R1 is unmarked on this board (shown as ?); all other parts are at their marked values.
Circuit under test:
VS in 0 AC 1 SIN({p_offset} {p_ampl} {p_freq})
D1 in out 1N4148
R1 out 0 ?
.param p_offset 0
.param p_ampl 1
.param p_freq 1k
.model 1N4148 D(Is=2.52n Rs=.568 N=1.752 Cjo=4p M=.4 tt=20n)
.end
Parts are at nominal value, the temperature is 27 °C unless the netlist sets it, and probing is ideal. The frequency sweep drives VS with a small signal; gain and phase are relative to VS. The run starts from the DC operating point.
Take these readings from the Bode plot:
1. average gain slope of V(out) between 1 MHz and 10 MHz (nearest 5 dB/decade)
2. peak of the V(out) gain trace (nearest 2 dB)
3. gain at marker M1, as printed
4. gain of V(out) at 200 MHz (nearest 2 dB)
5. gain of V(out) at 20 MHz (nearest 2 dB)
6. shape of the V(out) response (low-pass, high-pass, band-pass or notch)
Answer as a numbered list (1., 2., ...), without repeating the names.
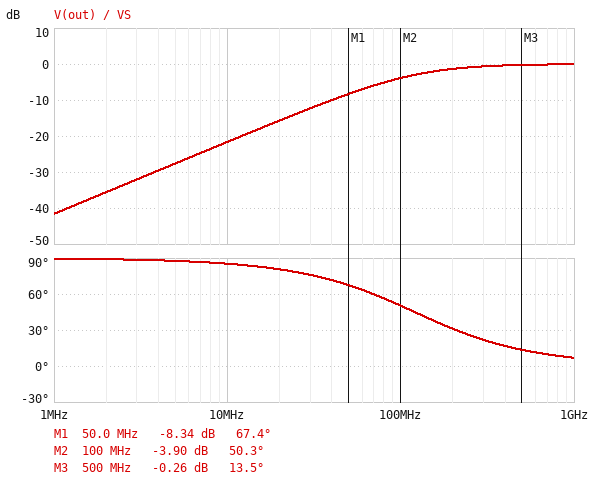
1. 20 dB/decade
2. 0 dB
3. -8.34 dB
4. -2 dB
5. -16 dB
6. high-pass
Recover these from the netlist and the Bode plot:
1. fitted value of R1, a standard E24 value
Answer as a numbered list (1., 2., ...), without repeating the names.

1. 330 Ω
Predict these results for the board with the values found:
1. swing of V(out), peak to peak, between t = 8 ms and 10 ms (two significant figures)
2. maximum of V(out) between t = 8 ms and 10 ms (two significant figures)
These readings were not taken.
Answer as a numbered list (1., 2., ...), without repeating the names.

1. 410 mV
2. 410 mV
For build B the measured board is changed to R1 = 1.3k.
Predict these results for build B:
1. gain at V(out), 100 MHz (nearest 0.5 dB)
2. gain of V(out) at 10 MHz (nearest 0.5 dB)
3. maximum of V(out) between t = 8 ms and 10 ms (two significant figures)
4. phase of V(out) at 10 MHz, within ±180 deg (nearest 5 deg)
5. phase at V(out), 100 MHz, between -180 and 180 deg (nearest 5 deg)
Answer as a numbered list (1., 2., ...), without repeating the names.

1. -0.5 dB
2. -10.0 dB
3. 460 mV
4. 70 deg
5. 15 deg
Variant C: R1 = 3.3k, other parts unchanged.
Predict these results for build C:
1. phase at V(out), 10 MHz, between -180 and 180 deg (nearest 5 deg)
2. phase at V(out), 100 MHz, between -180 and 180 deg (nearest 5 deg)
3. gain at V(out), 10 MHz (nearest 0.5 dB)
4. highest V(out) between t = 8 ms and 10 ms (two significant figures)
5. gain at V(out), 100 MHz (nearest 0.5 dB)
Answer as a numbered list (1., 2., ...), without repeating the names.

1. 50 deg
2. 5 deg
3. -4.0 dB
4. 500 mV
5. 0 dB
